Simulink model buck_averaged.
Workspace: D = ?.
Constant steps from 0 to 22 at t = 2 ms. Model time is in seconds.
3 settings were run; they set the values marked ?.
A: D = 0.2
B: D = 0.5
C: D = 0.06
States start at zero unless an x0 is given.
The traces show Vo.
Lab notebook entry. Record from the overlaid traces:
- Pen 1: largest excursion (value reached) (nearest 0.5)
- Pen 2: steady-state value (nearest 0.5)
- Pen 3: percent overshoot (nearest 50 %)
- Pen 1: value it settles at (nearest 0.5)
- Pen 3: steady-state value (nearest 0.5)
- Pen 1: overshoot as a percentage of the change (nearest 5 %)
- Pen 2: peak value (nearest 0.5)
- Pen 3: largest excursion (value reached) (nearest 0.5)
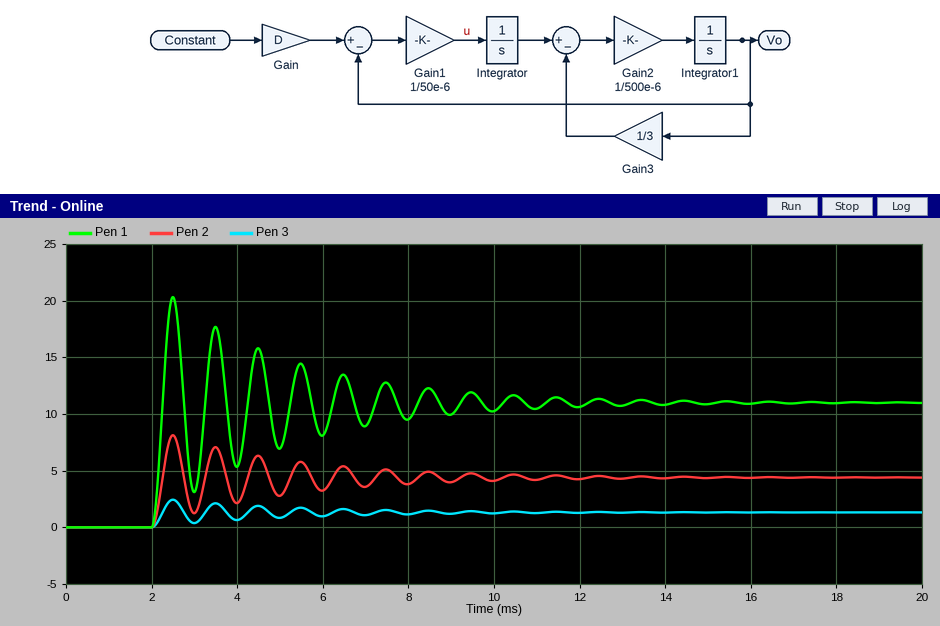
20.5
4.5
100 %
11.0
1.5
85 %
8.0
2.5
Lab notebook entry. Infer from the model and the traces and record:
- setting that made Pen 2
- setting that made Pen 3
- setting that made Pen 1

A
C
B
